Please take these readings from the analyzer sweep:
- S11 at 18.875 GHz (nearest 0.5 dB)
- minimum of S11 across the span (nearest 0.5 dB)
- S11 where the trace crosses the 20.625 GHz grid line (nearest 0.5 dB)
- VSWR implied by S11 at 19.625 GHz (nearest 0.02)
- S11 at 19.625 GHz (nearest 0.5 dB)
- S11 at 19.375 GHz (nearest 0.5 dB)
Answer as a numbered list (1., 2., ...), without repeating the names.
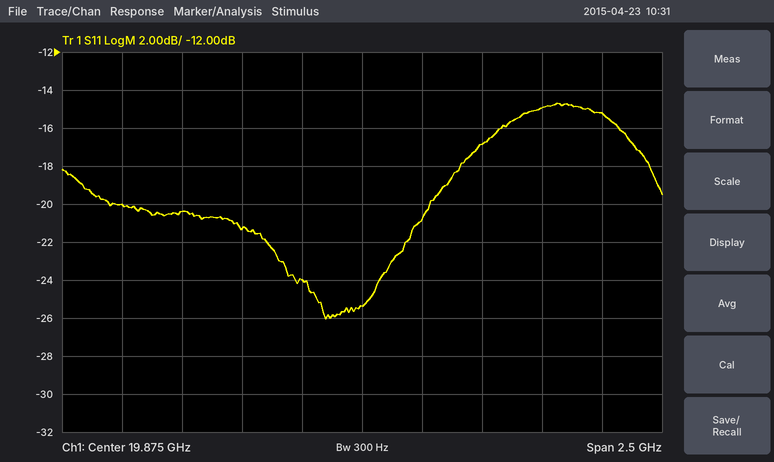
1. -20.0 dB
2. -26.0 dB
3. -15.0 dB
4. 1.14
5. -24.0 dB
6. -21.5 dB
